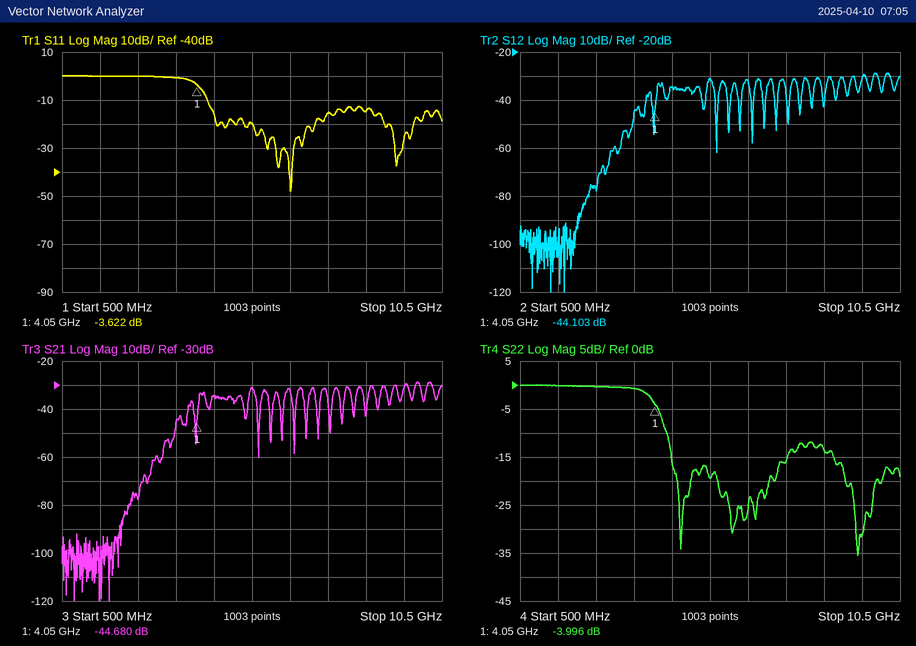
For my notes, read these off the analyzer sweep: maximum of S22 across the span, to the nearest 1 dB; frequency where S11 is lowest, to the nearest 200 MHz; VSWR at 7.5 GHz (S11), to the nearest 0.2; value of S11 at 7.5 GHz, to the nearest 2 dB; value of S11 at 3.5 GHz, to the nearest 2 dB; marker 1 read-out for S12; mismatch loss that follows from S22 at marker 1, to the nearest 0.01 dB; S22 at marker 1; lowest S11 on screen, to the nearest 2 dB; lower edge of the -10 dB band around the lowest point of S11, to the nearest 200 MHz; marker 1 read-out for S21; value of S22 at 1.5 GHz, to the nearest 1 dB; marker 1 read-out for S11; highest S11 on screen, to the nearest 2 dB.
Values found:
0 dB
6.6 GHz
1.4
-16 dB
0 dB
-44.103 dB
2.21 dB
-3.996 dB
-48 dB
4.4 GHz
-44.680 dB
0 dB
-3.622 dB
0 dB
